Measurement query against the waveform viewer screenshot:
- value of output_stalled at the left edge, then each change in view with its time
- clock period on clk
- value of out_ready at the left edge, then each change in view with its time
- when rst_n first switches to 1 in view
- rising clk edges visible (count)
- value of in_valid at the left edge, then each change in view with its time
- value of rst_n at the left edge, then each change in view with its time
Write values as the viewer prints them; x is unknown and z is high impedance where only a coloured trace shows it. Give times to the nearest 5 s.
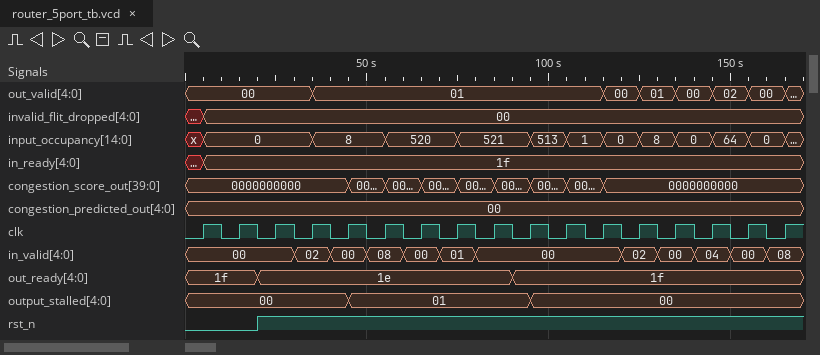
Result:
00, 01 at 45 s, 00 at 95 s
10 s
1f, 1e at 20 s, 1f at 90 s
20 s
17
00, 02 at 30 s, 00 at 40 s, 08 at 50 s, 00 at 60 s, 01 at 70 s, 00 at 80 s, 02 at 120 s, 00 at 130 s, 04 at 140 s, 00 at 150 s, 08 at 160 s
0, 1 at 20 s
